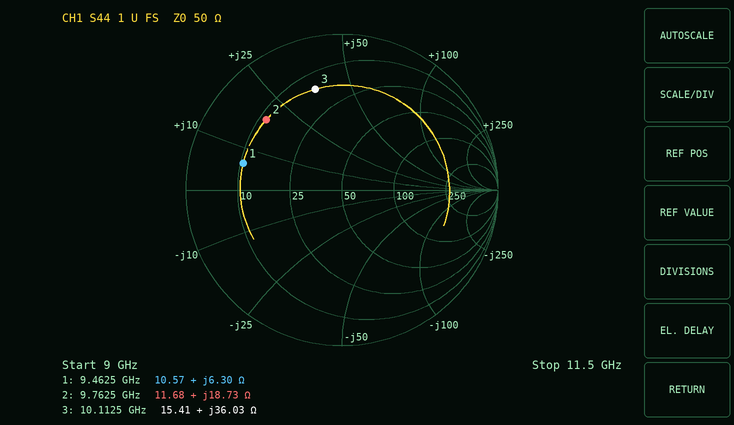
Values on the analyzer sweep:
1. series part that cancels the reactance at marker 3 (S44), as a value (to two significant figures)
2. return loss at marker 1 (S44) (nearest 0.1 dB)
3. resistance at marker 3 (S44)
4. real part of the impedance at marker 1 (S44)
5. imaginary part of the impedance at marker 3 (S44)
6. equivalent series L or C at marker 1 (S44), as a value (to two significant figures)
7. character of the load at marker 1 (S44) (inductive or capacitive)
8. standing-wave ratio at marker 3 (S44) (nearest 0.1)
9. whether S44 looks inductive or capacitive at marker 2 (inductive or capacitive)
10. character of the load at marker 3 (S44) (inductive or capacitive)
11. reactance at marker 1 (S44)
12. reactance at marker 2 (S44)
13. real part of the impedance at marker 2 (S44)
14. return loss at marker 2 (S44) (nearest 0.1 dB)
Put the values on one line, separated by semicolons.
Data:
440 fF; 3.7 dB; 15.41 Ω; 10.57 Ω; +36.03 Ω; 110 pH; inductive; 5.0; inductive; inductive; +6.30 Ω; +18.73 Ω; 11.68 Ω; 3.6 dB
